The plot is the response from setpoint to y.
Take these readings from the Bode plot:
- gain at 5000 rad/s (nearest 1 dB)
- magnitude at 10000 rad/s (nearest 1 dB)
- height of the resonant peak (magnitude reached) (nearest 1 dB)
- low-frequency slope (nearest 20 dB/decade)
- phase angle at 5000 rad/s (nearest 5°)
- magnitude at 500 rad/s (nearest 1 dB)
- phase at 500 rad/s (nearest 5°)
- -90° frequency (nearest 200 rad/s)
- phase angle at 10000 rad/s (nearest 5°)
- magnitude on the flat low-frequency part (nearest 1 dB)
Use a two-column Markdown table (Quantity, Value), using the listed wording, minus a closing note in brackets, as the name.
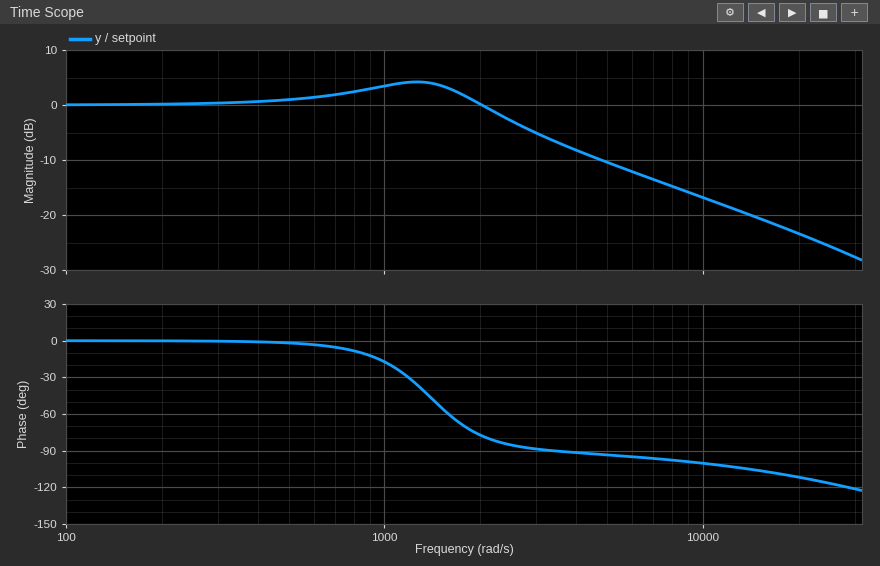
| Quantity | Value |
|---|---|
| gain at 5000 rad/s | -10 dB |
| magnitude at 10000 rad/s | -17 dB |
| height of the resonant peak (magnitude reached) | 4 dB |
| low-frequency slope | 0 dB/decade |
| phase angle at 5000 rad/s | -95° |
| magnitude at 500 rad/s | 1 dB |
| phase at 500 rad/s | 0° |
| -90° frequency | 3400 rad/s |
| phase angle at 10000 rad/s | -100° |
| magnitude on the flat low-frequency part | 0 dB |
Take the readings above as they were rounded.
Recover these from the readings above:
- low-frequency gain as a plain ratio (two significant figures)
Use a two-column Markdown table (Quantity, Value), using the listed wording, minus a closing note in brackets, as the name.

| Quantity | Value |
|---|---|
| low-frequency gain as a plain ratio | 1.0 |
